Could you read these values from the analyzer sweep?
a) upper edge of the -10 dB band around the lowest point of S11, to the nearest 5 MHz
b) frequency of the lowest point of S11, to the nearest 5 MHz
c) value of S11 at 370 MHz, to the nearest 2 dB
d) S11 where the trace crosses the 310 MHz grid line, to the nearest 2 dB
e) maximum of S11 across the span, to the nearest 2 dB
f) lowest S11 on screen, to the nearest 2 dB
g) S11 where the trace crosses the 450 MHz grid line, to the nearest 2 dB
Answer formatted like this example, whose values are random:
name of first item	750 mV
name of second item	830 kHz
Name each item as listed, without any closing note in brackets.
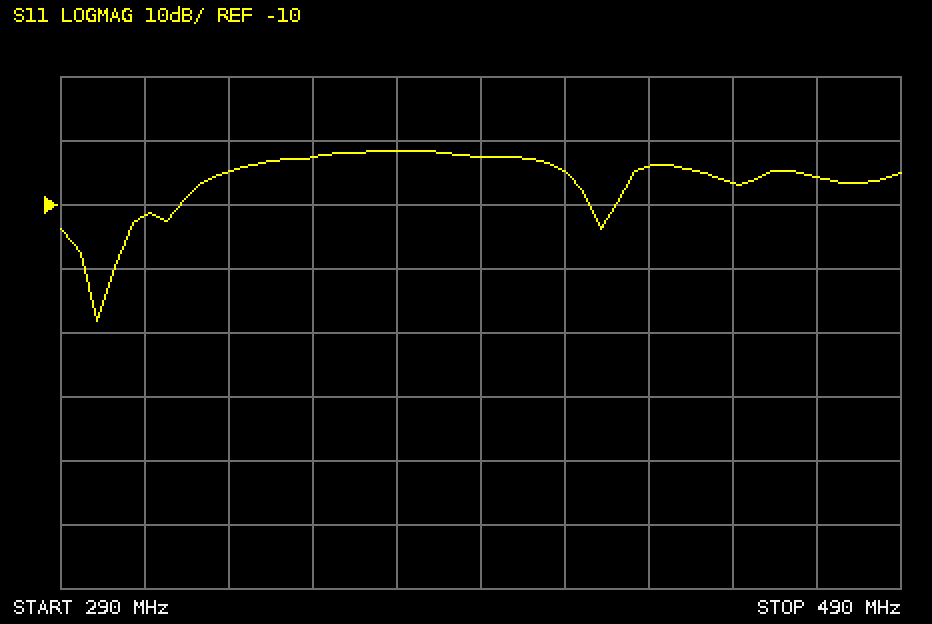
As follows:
upper edge of the -10 dB band around the lowest point of S11, to the nearest 5 MHz	320 MHz
frequency of the lowest point of S11, to the nearest 5 MHz	300 MHz
value of S11 at 370 MHz, to the nearest 2 dB	-2 dB
S11 where the trace crosses the 310 MHz grid line, to the nearest 2 dB	-12 dB
maximum of S11 across the span, to the nearest 2 dB	-2 dB
lowest S11 on screen, to the nearest 2 dB	-28 dB
S11 where the trace crosses the 450 MHz grid line, to the nearest 2 dB	-6 dB
